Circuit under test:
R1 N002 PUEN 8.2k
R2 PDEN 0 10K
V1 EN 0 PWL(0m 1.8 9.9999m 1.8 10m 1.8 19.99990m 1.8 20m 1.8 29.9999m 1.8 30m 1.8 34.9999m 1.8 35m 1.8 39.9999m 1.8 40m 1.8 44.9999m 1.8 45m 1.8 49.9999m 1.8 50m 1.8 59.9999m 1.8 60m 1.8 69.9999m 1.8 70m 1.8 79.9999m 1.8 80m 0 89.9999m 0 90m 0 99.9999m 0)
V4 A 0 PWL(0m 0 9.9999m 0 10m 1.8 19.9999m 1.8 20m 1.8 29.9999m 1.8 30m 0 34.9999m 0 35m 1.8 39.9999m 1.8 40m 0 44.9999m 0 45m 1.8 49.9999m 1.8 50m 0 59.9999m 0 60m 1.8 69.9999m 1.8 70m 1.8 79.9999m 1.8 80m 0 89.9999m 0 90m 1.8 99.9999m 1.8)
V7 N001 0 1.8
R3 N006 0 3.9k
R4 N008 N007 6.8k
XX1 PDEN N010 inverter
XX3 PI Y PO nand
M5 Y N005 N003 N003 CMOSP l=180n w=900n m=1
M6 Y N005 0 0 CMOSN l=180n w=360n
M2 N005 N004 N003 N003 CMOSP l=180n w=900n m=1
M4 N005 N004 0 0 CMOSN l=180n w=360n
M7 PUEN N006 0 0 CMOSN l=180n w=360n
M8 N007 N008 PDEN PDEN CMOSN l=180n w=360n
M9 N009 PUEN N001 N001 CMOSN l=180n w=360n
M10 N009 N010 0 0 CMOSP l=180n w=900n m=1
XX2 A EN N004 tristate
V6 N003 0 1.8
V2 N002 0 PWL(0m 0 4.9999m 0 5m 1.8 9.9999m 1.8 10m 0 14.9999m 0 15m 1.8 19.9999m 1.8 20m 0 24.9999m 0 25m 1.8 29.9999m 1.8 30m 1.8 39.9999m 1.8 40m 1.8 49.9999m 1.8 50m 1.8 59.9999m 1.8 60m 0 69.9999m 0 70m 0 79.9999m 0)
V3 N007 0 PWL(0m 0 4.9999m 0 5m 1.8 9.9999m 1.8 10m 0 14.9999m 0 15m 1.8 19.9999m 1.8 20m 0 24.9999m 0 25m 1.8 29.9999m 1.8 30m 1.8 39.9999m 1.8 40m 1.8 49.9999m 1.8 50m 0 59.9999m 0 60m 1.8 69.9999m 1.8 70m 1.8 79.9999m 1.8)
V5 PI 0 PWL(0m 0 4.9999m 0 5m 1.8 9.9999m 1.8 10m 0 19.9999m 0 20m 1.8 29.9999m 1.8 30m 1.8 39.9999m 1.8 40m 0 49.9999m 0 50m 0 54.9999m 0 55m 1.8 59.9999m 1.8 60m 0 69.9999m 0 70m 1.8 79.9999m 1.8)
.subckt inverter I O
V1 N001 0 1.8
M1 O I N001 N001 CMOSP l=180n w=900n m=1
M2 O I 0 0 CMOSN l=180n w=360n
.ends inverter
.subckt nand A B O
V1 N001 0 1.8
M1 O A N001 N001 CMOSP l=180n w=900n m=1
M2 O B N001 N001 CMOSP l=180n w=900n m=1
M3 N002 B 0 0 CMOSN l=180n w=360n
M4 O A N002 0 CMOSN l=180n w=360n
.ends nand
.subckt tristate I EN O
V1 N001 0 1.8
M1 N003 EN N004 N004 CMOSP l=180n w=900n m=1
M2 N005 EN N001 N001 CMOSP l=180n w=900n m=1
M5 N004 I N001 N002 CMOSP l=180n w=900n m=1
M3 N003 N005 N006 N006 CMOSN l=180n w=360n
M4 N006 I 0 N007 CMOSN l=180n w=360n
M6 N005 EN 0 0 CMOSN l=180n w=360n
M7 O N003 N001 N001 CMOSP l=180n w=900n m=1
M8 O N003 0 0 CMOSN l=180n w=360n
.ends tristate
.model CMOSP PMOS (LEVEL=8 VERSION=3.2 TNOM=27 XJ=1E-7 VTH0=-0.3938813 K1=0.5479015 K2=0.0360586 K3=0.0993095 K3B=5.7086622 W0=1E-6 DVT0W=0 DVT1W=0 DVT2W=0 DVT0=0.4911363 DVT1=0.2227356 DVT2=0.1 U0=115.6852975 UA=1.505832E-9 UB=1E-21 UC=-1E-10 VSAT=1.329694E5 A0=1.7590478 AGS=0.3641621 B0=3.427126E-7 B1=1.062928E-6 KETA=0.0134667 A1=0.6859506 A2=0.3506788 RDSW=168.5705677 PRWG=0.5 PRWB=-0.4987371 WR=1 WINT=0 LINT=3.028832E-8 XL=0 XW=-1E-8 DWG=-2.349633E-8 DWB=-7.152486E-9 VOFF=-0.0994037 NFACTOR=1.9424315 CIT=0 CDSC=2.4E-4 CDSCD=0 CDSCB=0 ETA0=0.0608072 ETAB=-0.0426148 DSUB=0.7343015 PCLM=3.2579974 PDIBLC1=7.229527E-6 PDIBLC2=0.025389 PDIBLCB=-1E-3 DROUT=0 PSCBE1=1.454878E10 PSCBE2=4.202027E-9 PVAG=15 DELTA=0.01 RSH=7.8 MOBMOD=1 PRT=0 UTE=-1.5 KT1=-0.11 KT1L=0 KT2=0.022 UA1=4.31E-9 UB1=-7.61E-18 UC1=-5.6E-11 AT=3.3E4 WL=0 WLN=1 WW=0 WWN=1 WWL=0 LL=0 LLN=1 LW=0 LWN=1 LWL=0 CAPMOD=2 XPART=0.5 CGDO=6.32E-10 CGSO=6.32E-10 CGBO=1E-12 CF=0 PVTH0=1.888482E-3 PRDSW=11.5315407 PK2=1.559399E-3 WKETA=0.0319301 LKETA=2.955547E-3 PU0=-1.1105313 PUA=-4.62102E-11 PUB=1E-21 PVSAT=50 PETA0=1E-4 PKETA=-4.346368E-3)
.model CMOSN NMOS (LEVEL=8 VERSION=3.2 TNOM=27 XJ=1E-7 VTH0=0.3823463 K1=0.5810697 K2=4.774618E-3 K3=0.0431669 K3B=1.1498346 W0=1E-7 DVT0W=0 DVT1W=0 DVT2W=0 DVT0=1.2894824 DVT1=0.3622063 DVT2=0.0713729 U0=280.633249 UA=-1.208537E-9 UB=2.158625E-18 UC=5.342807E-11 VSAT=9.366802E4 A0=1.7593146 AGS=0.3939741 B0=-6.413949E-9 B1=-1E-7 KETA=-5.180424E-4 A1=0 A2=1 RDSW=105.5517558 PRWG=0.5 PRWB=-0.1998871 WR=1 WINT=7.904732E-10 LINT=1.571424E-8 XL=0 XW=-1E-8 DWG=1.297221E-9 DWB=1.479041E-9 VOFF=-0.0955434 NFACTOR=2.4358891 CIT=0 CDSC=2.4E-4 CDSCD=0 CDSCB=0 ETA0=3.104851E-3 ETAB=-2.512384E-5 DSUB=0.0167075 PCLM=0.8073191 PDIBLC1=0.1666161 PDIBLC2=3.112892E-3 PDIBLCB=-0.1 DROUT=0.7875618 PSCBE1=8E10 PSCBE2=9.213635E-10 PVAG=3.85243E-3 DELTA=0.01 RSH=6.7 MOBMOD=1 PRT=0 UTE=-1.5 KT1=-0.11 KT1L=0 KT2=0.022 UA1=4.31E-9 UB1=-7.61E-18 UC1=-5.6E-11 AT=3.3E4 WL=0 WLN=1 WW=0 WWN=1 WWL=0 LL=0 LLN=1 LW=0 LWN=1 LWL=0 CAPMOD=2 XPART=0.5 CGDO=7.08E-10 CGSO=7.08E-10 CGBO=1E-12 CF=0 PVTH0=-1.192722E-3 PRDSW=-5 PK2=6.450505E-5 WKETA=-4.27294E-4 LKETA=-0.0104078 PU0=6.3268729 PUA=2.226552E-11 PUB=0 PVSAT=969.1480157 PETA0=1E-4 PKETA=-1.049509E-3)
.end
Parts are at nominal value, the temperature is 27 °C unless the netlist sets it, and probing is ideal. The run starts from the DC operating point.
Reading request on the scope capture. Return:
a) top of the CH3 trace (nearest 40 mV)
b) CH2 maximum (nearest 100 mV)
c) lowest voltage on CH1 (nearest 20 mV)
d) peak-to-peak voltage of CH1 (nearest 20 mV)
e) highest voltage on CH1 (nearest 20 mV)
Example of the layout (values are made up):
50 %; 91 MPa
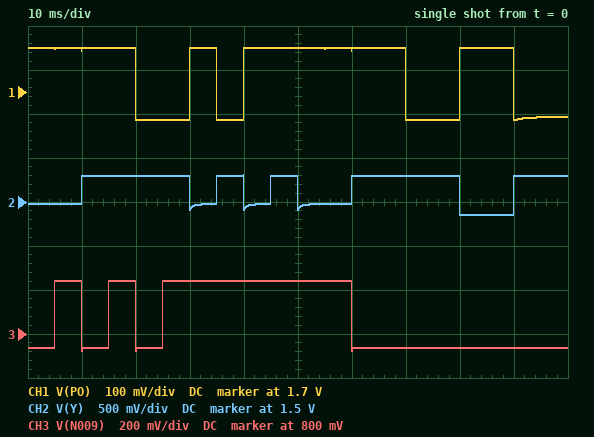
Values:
1.04 V; 1.8 V; 1.64 V; 160 mV; 1.80 V
